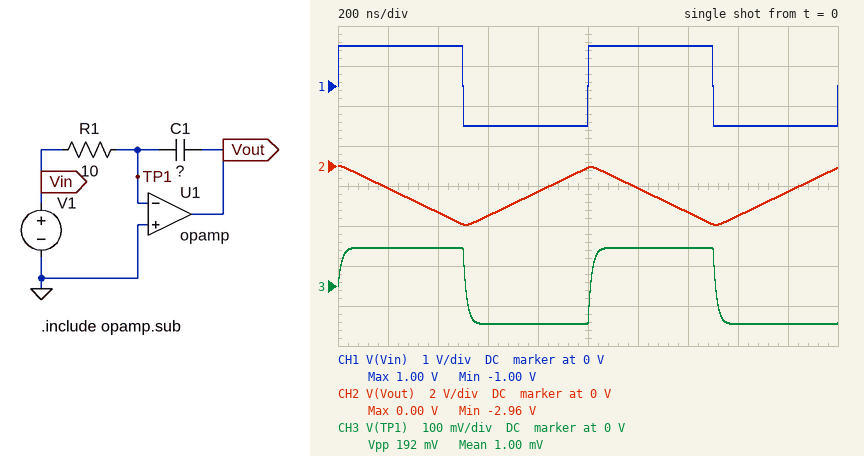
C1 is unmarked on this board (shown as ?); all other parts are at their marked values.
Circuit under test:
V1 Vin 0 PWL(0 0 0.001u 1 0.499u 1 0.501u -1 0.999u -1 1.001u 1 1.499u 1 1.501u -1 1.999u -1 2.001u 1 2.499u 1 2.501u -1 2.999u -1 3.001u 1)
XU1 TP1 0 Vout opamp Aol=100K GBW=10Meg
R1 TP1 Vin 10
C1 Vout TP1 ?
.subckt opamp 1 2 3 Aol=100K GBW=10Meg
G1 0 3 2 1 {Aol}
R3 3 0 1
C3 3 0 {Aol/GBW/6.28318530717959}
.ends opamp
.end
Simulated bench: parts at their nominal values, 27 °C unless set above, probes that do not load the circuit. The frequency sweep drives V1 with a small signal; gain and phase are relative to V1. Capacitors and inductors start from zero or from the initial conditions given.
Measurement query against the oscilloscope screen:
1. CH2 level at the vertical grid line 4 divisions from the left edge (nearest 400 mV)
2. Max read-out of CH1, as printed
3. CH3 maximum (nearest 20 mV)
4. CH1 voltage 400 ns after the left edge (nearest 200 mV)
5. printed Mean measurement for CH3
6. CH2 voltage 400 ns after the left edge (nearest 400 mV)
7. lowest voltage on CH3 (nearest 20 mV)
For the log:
-1.2 V
1.00 V
100 mV
1.0 V
1.00 mV
-2.4 V
-100 mV
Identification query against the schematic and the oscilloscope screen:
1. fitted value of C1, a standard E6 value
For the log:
15 nF
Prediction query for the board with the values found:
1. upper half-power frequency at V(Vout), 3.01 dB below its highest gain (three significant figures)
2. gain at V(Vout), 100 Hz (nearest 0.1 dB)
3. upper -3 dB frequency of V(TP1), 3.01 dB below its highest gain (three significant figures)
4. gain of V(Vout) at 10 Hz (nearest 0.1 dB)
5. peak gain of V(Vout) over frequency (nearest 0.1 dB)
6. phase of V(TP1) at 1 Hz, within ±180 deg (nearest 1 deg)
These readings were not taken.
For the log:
9.59 Hz
79.6 dB
9.68 Hz
96.8 dB
100.0 dB
-5 deg
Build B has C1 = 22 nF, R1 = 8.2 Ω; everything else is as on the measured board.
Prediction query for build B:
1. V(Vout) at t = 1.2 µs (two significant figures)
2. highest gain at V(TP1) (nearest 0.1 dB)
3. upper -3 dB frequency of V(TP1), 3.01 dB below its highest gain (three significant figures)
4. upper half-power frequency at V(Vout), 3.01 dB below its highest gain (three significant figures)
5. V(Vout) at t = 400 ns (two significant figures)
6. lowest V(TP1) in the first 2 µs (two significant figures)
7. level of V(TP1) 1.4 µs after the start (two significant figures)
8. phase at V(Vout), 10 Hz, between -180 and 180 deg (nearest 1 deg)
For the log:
-940 mV
0 dB
8.16 Hz
8.11 Hz
-2.0 V
-81 mV
81 mV
129 deg
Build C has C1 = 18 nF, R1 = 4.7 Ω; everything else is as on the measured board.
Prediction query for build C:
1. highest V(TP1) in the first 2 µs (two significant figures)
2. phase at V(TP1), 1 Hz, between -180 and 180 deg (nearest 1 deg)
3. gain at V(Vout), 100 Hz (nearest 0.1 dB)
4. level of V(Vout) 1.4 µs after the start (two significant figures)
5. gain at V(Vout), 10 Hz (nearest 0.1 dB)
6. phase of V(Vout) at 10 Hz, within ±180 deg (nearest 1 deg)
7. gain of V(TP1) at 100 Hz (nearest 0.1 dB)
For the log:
160 mV
-3 deg
83.9 dB
-3.8 V
98.5 dB
148 deg
-13.1 dB
